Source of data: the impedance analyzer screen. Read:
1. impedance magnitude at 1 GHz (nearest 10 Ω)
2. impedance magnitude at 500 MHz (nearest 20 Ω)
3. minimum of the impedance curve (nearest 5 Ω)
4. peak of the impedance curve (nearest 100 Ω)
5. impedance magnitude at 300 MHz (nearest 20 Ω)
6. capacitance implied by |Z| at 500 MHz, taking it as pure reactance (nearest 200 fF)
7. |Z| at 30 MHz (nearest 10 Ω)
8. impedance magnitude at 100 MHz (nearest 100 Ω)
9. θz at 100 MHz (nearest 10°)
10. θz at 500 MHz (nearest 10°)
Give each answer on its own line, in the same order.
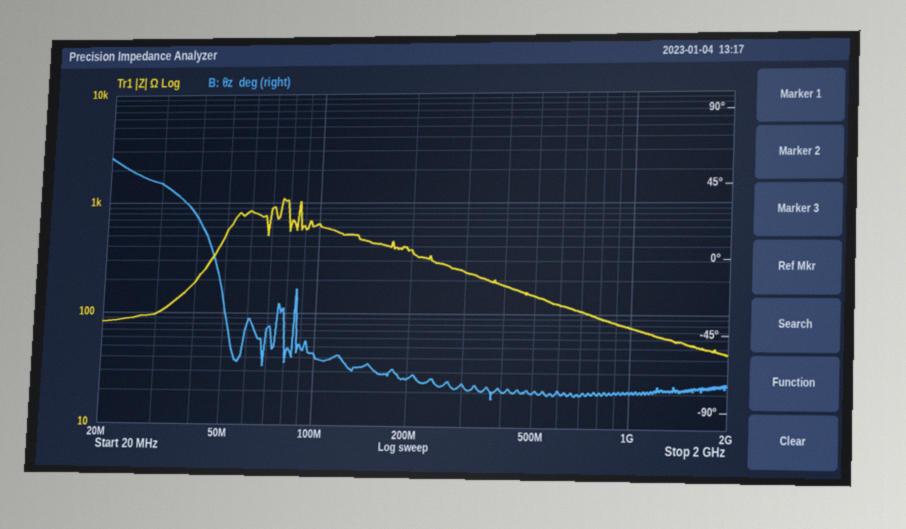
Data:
80 Ω
140 Ω
45 Ω
1.1 kΩ
240 Ω
2.2 pF
100 Ω
600 Ω
-60°
-80°
